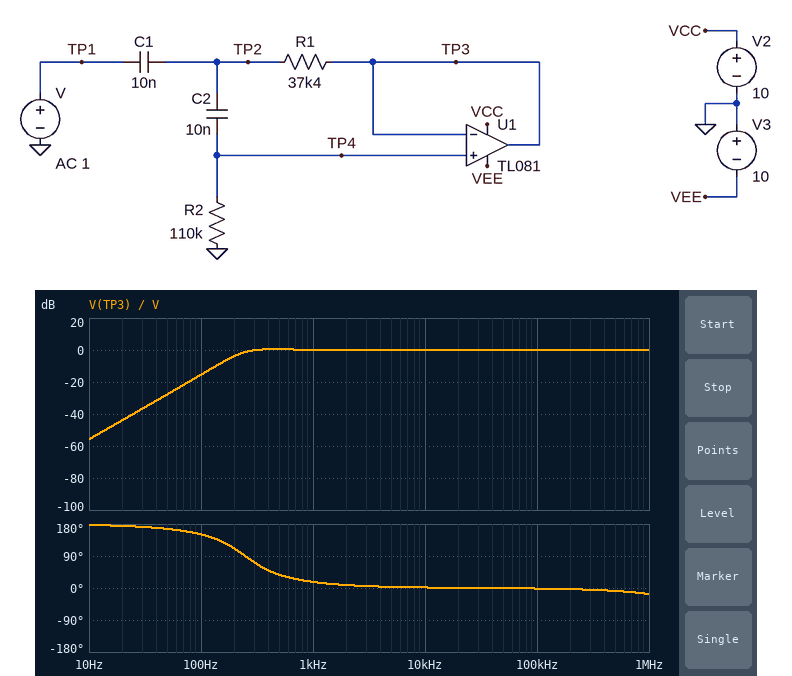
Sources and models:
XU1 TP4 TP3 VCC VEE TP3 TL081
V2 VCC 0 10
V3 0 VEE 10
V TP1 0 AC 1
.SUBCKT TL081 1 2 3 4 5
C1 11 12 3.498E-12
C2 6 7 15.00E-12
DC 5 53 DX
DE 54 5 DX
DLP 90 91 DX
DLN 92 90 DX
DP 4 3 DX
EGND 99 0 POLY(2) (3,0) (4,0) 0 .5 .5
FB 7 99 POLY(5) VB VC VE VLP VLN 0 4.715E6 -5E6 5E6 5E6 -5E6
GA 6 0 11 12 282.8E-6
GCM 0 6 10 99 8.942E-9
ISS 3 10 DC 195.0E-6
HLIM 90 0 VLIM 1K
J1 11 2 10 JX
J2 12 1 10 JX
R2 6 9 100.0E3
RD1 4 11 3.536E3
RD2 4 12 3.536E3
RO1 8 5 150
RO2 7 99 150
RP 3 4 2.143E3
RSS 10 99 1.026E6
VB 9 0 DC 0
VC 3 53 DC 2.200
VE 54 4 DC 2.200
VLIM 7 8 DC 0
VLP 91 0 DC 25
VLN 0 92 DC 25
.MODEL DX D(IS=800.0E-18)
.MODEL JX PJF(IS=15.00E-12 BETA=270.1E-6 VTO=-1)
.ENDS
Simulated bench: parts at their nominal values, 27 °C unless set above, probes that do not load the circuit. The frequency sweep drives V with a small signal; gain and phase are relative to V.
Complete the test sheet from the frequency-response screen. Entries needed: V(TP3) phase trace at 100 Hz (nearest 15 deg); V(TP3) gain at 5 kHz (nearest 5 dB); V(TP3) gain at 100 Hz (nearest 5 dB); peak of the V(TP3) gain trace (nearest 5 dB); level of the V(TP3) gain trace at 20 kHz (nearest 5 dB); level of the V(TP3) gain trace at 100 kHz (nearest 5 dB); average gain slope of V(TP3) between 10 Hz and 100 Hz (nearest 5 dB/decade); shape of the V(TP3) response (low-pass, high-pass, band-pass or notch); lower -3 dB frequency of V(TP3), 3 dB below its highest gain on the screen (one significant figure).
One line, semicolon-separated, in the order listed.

150 deg; 0 dB; -15 dB; 0 dB; 0 dB; 0 dB; 40 dB/decade; high-pass; 200 Hz
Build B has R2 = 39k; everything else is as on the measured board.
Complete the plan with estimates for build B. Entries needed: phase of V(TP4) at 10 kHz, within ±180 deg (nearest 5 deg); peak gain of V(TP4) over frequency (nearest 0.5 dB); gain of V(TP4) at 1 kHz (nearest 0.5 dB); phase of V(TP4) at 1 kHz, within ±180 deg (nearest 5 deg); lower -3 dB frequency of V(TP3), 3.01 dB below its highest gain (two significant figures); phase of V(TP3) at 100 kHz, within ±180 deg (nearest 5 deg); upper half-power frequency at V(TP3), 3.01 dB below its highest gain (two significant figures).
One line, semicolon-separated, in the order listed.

5 deg; 0 dB; -1.5 dB; 45 deg; 630 Hz; 0 deg; 4.8 MHz
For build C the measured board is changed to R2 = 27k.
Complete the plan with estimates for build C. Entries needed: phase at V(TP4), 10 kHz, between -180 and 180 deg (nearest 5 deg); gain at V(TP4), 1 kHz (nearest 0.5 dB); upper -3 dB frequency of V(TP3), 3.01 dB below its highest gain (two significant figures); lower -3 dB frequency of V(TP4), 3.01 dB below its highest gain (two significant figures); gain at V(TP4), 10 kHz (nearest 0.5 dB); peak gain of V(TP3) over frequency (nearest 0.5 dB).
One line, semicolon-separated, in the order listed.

5 deg; -3.0 dB; 4.8 MHz; 980 Hz; 0 dB; 0 dB
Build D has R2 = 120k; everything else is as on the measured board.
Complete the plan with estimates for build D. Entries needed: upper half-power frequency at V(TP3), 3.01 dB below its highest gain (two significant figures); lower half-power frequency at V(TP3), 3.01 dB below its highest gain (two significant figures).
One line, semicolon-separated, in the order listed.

4.5 MHz; 210 Hz
